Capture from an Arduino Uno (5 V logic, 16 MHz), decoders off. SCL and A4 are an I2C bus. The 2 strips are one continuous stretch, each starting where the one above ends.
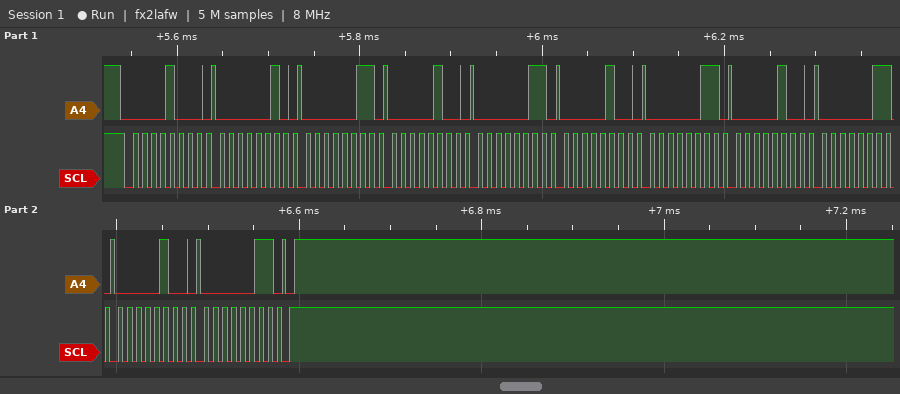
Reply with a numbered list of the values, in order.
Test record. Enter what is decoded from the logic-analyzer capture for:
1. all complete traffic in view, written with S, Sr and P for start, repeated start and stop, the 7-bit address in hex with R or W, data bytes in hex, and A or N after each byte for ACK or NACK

1. S 04W A 02 A 03 A 04 A 03 A 04 A 03 A 04 A 03 A 04 A 03 A P
